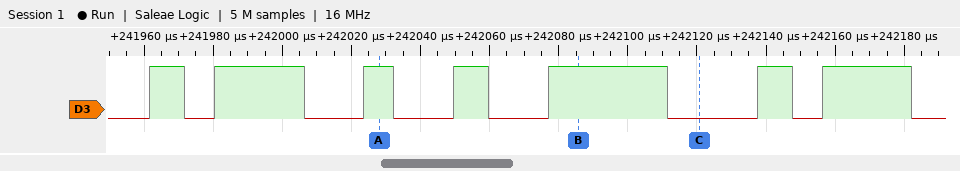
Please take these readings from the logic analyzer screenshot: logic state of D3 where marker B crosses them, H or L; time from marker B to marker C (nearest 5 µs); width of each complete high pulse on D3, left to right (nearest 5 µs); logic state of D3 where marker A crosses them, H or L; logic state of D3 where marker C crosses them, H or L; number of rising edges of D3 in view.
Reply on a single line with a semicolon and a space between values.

D3=H; 35 µs; 10 µs, 25 µs, 10 µs, 10 µs, 35 µs, 10 µs, 25 µs; D3=H; D3=L; 7
